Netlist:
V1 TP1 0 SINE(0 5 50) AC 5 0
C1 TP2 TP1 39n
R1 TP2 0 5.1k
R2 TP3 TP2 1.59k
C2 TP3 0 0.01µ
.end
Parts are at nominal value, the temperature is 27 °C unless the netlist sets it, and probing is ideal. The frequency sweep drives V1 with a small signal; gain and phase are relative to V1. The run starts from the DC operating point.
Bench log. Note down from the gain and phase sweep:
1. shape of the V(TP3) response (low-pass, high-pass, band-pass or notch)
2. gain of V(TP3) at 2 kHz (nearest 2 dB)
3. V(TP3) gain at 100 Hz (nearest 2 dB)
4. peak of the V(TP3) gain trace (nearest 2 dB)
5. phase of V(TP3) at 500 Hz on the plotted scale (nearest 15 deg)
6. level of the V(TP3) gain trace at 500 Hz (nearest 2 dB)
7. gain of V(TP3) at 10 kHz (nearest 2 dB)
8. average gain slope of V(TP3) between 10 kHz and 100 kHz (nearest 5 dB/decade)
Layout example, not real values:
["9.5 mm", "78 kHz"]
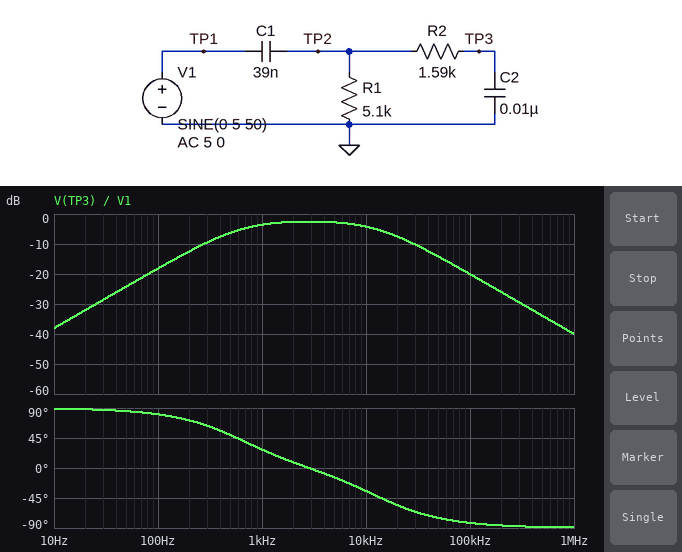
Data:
["band-pass", "-2 dB", "-18 dB", "-2 dB", "45 deg", "-6 dB", "-4 dB", "-15 dB/decade"]
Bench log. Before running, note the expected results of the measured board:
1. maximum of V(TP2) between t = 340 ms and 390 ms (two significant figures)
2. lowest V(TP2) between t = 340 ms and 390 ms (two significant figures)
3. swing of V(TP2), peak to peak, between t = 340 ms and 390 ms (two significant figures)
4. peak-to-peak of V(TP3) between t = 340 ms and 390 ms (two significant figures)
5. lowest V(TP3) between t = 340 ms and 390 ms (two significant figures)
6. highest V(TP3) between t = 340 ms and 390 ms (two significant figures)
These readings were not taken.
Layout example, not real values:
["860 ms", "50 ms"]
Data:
["310 mV", "-310 mV", "620 mV", "620 mV", "-310 mV", "310 mV"]
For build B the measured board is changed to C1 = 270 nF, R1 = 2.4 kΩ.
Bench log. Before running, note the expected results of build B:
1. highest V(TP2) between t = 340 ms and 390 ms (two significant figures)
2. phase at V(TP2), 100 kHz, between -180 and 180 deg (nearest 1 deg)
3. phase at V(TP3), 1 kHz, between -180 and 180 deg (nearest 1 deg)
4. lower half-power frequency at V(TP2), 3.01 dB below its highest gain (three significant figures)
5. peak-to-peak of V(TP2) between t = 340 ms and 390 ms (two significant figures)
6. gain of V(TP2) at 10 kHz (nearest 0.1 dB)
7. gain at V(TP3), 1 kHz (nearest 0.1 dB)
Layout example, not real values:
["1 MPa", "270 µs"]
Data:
["1.0 V", "0 deg", "8 deg", "256 Hz", "2.0 V", "-0.2 dB", "-0.6 dB"]
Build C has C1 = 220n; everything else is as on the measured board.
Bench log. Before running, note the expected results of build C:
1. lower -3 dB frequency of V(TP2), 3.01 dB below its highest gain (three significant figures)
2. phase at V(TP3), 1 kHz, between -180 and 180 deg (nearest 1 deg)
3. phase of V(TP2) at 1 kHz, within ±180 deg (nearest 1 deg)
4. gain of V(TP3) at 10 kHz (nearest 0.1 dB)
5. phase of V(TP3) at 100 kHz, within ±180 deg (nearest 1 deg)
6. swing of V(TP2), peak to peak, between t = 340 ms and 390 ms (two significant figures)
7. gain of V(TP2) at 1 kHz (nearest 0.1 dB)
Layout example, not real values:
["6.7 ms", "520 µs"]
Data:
["149 Hz", "2 deg", "8 deg", "-3.2 dB", "-84 deg", "3.3 V", "-0.5 dB"]
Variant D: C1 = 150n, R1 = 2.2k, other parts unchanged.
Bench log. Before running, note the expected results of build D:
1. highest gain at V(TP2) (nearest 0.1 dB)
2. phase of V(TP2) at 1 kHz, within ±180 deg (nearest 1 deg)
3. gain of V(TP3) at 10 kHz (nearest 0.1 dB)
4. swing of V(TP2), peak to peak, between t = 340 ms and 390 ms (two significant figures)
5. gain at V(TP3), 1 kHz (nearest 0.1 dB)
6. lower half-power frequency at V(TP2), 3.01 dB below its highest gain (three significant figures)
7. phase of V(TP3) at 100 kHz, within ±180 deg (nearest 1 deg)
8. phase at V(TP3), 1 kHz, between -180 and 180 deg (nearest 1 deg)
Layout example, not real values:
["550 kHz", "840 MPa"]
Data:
["0 dB", "25 deg", "-3.3 dB", "1.0 V", "-1.4 dB", "521 Hz", "-84 deg", "19 deg"]
